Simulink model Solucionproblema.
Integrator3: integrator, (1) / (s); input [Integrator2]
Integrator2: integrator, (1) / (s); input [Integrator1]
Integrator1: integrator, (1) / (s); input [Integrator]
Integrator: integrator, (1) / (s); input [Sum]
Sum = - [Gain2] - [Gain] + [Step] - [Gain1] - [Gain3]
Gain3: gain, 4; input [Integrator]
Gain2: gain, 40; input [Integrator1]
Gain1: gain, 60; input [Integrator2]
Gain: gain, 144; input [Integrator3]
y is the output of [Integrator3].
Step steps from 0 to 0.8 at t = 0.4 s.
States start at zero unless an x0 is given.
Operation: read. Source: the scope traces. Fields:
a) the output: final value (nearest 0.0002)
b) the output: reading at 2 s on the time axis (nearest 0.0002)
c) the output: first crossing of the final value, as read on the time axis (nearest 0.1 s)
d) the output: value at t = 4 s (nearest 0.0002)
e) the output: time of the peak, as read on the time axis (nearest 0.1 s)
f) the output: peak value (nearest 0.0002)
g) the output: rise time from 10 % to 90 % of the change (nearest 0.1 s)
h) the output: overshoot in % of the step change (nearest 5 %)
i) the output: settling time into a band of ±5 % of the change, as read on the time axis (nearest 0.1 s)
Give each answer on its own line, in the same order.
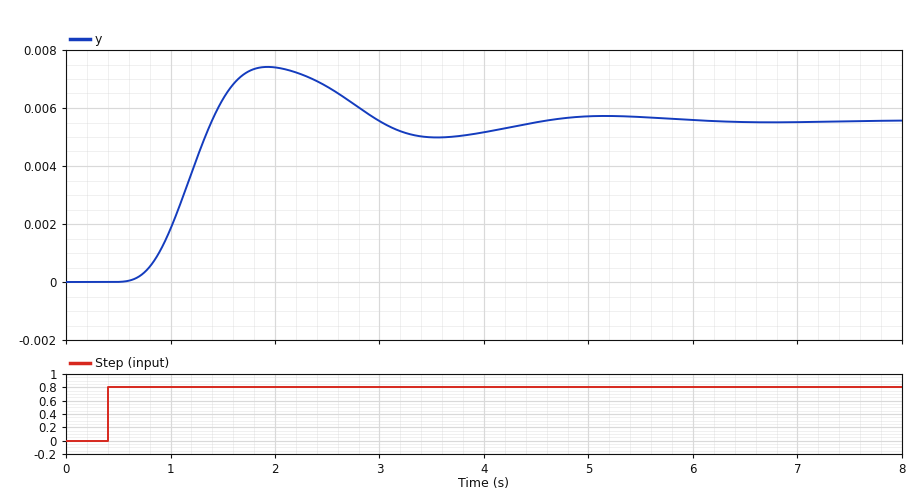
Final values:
0.0056
0.0074
1.4 s
0.0052
1.9 s
0.0074
0.5 s
35 %
4.2 s
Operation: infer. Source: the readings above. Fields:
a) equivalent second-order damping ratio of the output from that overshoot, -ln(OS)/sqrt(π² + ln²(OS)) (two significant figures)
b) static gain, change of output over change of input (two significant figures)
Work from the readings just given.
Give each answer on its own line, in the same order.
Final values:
0.32
0.0070
